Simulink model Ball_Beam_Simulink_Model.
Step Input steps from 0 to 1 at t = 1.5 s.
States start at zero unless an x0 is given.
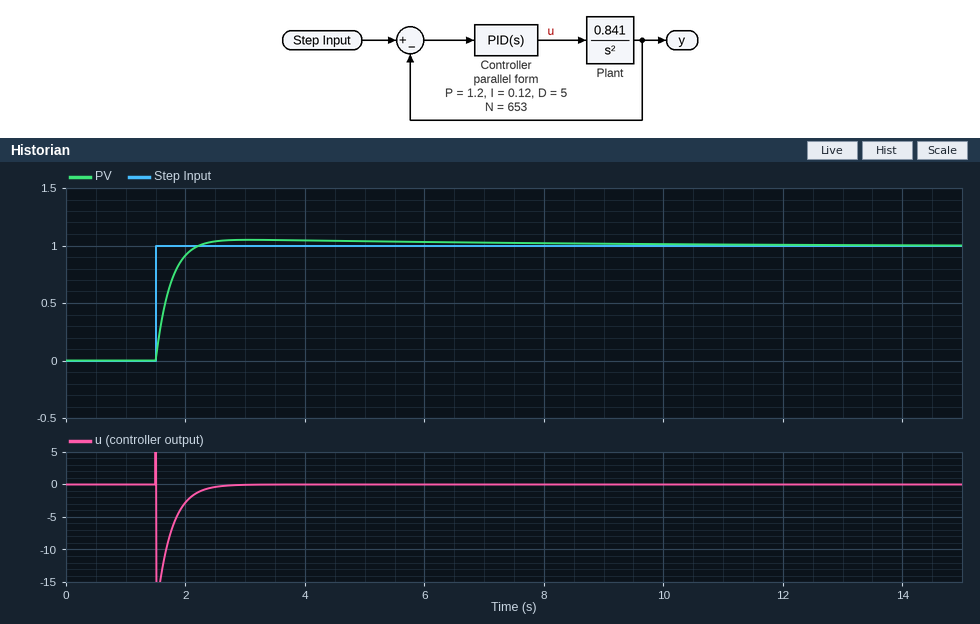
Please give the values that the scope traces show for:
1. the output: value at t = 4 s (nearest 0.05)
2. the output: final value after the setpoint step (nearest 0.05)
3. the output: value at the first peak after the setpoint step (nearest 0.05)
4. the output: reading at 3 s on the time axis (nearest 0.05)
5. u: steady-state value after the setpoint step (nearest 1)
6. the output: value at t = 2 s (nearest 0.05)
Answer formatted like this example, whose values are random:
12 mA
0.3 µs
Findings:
1.05
1.00
1.05
1.05
0
0.90
